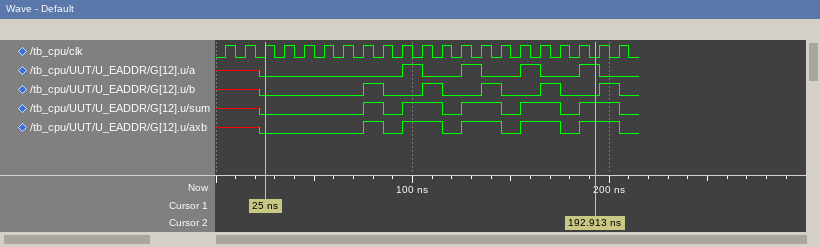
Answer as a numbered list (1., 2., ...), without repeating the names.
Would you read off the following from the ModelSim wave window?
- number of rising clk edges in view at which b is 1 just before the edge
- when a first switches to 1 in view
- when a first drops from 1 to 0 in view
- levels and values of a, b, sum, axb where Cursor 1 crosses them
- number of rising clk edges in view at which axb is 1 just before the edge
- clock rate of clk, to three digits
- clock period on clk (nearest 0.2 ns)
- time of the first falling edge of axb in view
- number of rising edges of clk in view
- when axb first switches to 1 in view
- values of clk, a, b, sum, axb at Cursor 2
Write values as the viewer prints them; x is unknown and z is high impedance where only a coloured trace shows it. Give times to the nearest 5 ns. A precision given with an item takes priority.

1. 5
2. 95 ns
3. 105 ns
4. a=0, b=0, sum=0, axb=0
5. 9
6. 100 MHz
7. 10 ns
8. 85 ns
9. 21
10. 75 ns
11. clk=0, a=1, b=0, sum=1, axb=1
